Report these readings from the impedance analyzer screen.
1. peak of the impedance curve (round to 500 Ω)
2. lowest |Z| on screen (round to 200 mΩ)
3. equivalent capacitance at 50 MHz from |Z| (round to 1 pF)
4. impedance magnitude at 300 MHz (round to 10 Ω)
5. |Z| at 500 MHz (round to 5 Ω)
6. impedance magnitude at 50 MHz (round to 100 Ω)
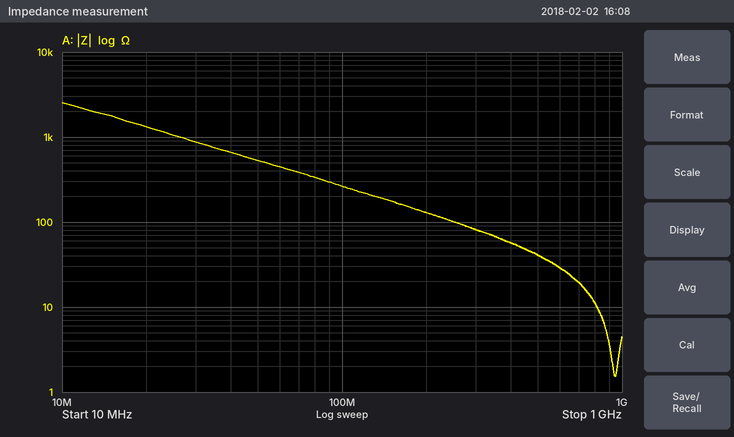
2.5 kΩ
1.6 Ω
6 pF
80 Ω
40 Ω
500 Ω
